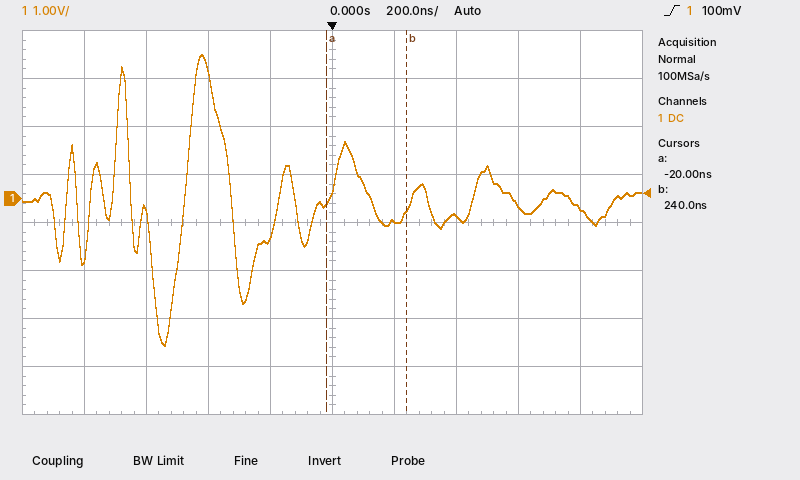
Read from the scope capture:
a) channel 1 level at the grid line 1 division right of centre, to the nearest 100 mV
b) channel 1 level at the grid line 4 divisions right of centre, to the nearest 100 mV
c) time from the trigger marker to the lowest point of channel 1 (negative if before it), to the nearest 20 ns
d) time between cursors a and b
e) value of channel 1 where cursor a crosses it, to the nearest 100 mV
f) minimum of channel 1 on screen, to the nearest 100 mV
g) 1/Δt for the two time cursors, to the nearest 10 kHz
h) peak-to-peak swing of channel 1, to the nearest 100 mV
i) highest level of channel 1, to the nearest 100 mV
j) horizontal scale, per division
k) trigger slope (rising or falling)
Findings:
-500 mV
-200 mV
-540 ns
260 ns
-100 mV
-3.1 V
3.85 MHz
6.1 V
3.0 V
200 ns
rising
